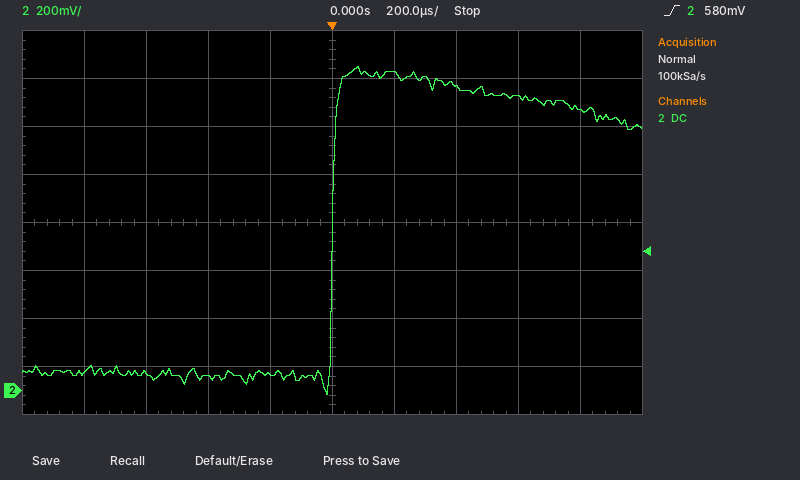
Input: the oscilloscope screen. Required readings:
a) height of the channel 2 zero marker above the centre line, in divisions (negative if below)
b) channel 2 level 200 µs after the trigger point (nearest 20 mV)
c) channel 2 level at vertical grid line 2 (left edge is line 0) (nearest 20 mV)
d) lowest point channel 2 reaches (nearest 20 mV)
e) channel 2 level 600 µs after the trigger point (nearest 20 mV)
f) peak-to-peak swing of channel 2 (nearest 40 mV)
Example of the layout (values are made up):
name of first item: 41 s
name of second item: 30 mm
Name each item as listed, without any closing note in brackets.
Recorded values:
height of the channel 2 zero marker above the centre line, in divisions: -3.5 div
channel 2 level 200 µs after the trigger point: 1.32 V
channel 2 level at vertical grid line 2 (left edge is line 0): 80 mV
lowest point channel 2 reaches: -20 mV
channel 2 level 600 µs after the trigger point: 1.22 V
peak-to-peak swing of channel 2: 1.36 V
